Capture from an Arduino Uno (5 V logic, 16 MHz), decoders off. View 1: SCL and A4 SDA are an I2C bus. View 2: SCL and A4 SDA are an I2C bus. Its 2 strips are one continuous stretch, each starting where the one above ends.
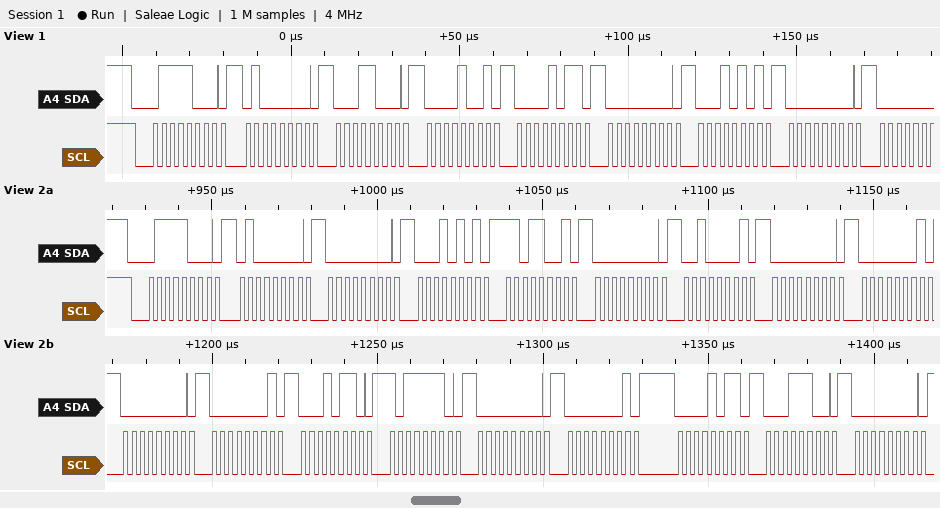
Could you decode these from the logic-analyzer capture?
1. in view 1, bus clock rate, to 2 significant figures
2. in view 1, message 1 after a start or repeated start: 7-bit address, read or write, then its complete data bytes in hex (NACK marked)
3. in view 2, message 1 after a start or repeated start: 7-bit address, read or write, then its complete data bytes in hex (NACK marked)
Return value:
400 kHz
0x3C write: 40 18 09 0B 00 15 00
0x3C write: 40 00 15 D9 00 21 00 01 00 01 16 BE 00 01 0B 1C 00
